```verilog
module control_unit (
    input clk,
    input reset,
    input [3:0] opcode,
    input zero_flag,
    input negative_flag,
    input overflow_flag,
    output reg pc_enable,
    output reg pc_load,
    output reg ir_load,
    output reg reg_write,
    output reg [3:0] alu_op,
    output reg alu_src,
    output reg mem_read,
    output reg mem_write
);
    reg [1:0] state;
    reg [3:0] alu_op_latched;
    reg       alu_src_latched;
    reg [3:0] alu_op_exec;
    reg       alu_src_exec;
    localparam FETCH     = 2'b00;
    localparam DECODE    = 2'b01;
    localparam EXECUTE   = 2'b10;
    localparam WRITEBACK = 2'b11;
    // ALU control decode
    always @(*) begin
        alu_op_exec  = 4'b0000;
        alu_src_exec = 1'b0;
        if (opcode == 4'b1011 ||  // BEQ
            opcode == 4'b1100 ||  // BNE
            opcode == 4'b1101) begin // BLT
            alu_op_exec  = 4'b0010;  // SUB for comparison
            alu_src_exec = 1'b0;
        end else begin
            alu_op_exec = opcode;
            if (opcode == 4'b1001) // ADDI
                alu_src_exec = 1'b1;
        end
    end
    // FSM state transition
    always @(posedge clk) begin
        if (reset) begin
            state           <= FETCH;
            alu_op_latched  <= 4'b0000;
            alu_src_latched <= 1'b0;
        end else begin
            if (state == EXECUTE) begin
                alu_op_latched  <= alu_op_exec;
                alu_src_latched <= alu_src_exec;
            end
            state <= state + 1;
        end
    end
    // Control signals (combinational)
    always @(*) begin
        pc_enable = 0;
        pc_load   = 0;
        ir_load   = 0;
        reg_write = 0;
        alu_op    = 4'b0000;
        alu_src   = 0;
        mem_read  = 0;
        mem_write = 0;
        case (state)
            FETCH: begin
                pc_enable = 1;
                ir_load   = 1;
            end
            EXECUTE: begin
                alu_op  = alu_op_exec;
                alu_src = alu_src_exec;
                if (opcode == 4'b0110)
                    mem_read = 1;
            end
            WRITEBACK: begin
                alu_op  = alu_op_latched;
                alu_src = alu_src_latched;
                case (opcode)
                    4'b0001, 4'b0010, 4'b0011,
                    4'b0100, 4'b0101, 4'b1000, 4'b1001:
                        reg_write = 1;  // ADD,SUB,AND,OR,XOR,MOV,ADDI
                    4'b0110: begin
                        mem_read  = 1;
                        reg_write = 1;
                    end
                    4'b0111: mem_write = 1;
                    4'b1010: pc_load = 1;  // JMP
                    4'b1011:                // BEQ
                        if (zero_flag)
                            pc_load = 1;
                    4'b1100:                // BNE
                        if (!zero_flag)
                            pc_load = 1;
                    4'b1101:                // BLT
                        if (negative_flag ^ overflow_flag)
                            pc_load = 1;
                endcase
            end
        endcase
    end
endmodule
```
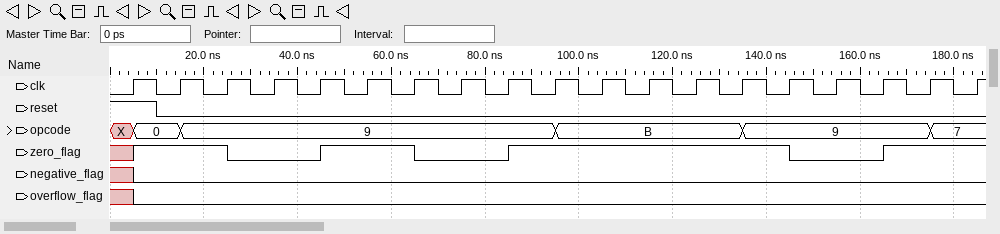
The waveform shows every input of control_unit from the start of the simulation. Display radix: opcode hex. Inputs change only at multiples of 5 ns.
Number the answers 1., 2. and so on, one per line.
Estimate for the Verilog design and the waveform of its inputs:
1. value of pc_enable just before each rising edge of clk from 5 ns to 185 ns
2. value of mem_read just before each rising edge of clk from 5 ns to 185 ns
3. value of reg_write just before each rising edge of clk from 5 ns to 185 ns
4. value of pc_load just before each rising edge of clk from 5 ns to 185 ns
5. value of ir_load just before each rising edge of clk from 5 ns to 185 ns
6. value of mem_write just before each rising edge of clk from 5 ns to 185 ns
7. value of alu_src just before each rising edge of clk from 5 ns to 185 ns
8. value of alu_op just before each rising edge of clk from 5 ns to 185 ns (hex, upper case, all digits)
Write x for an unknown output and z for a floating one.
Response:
1. x 1 0 0 0 1 0 0 0 1 0 0 0 1 0 0 0 1 0
2. x 0 0 0 0 0 0 0 0 0 0 0 0 0 0 0 0 0 0
3. x 0 0 0 1 0 0 0 1 0 0 0 0 0 0 0 1 0 0
4. x 0 0 0 0 0 0 0 0 0 0 0 1 0 0 0 0 0 0
5. x 1 0 0 0 1 0 0 0 1 0 0 0 1 0 0 0 1 0
6. x 0 0 0 0 0 0 0 0 0 0 0 0 0 0 0 0 0 0
7. x 0 0 1 1 0 0 1 1 0 0 0 0 0 0 1 1 0 0
8. x, 0, 0, 9, 9, 0, 0, 9, 9, 0, 0, 2, 2, 0, 0, 9, 9, 0, 0
